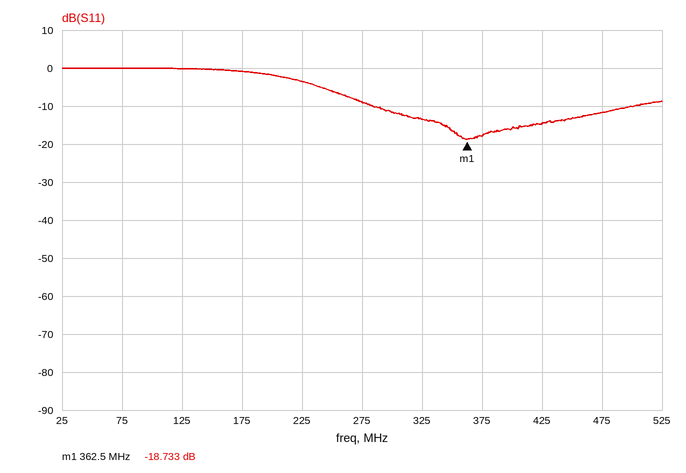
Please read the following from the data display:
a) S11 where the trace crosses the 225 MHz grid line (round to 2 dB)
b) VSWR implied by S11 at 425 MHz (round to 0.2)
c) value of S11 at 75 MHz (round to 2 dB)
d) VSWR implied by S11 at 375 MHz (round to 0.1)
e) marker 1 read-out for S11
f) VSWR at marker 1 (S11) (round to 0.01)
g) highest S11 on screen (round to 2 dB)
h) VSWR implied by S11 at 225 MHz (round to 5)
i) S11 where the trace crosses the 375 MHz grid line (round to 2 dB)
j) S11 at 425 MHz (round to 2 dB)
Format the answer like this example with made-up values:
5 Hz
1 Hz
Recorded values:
-4 dB
1.4
0 dB
1.3
-18.733 dB
1.26
0 dB
5
-18 dB
-14 dB
